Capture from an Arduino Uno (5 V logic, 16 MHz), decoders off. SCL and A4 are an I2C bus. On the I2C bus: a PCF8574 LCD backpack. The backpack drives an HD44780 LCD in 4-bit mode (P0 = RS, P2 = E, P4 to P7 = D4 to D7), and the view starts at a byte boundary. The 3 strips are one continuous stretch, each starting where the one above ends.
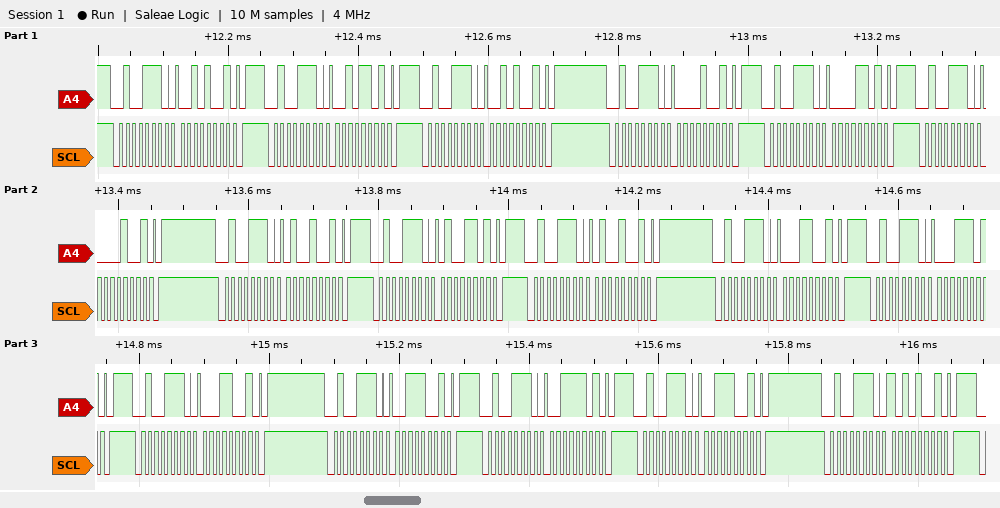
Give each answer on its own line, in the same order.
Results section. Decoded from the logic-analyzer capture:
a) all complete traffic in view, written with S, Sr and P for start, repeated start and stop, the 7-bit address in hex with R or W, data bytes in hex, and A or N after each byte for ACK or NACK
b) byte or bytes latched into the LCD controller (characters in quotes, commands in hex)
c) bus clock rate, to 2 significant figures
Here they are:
S 27W A 29 A P S 27W A 2D A P S 27W A 29 A P S 27W A 09 A P S 27W A 0D A P S 27W A 09 A P S 27W A 49 A P S 27W A 4D A P S 27W A 49 A P S 27W A 19 A P S 27W A 1D A P S 27W A 19 A P S 27W A 39 A P S 27W A 3D A P S 27W A 39 A P S 27W A A9 A P
' ' 'A'
100 kHz
